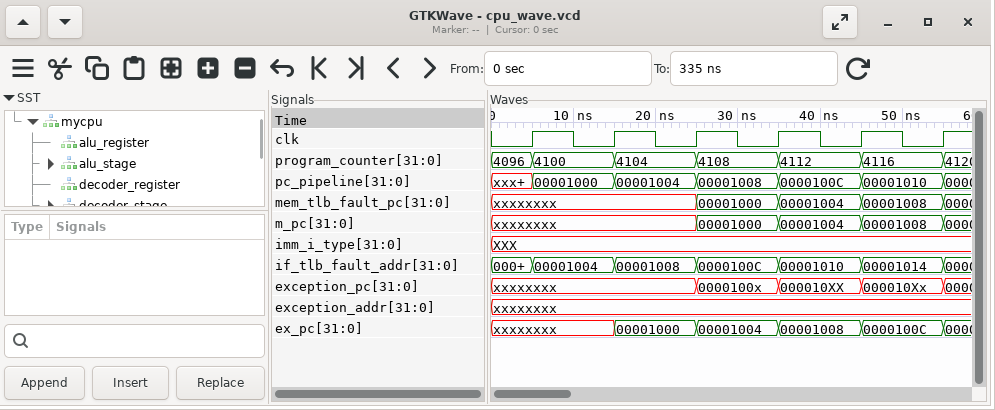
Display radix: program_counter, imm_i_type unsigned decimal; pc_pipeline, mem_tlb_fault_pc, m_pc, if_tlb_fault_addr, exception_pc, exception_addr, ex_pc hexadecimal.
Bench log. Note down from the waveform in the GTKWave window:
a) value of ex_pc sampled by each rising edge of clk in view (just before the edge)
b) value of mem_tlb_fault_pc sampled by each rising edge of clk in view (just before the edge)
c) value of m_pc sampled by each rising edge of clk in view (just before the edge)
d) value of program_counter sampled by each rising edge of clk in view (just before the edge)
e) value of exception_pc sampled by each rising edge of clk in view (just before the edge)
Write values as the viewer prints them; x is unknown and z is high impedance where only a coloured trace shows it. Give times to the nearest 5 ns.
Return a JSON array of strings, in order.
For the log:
["xxxxxxxx, xxxxxxxx, 00001000, 00001004, 00001008, 0000100C", "xxxxxxxx, xxxxxxxx, xxxxxxxx, 00001000, 00001004, 00001008", "xxxxxxxx, xxxxxxxx, xxxxxxxx, 00001000, 00001004, 00001008", "4096, 4100, 4104, 4108, 4112, 4116", "xxxxxxxx, xxxxxxxx, xxxxxxxx, 0000100x, 000010XX, 000010Xx"]
